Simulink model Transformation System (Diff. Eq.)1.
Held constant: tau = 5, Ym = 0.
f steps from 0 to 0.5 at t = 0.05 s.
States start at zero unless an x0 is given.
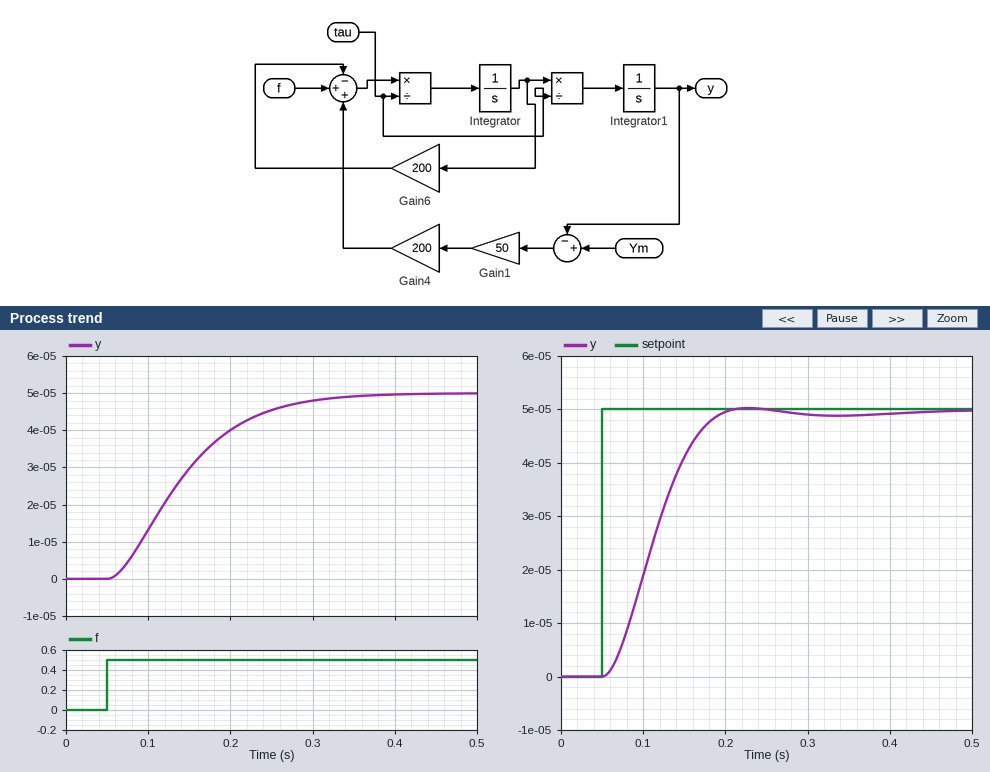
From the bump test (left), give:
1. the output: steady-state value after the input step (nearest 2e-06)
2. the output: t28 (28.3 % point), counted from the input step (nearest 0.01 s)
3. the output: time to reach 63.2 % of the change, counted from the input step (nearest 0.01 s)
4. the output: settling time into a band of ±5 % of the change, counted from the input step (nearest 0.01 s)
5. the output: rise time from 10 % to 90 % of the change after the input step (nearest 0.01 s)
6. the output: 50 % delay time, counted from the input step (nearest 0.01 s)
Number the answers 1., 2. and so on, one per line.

1. 0.000050
2. 0.05 s
3. 0.11 s
4. 0.24 s
5. 0.17 s
6. 0.08 s
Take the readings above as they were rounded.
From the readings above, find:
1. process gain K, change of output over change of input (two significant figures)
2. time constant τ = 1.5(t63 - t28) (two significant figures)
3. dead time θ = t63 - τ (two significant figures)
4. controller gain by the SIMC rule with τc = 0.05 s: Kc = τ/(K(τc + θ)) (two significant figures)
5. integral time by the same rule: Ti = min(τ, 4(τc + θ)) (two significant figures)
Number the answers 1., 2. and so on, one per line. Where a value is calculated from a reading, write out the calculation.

1. (5e-05 - 0) / 0.5 = 0.00010
2. 1.5 × (0.11 - 0.05) = 0.090 s
3. 0.11 - 0.09 = 0.020 s
4. 0.09 / (0.0001 × (0.05 + 0.02)) = 13000
5. min(0.09, 4 × (0.05 + 0.02)) = 0.090 s
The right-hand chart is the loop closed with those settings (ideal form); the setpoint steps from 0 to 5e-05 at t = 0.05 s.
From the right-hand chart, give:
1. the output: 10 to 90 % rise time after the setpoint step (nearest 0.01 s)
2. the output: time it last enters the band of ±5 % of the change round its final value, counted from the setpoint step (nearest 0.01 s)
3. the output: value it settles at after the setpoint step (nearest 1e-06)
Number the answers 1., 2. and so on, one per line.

1. 0.09 s
2. 0.13 s
3. 0.000050
